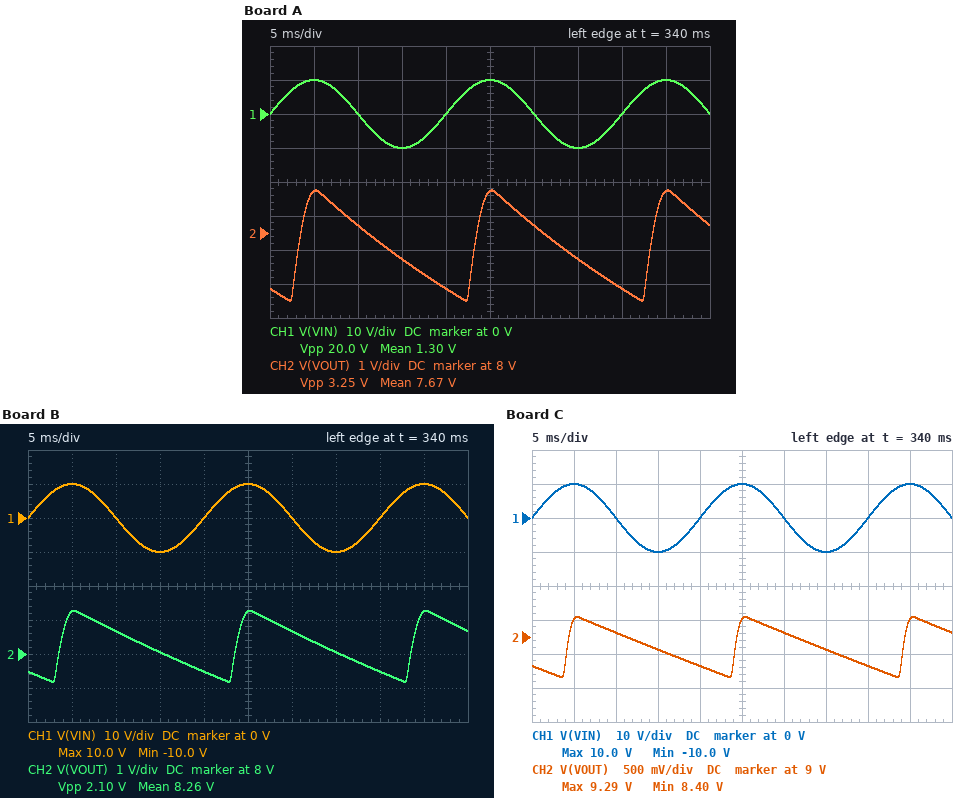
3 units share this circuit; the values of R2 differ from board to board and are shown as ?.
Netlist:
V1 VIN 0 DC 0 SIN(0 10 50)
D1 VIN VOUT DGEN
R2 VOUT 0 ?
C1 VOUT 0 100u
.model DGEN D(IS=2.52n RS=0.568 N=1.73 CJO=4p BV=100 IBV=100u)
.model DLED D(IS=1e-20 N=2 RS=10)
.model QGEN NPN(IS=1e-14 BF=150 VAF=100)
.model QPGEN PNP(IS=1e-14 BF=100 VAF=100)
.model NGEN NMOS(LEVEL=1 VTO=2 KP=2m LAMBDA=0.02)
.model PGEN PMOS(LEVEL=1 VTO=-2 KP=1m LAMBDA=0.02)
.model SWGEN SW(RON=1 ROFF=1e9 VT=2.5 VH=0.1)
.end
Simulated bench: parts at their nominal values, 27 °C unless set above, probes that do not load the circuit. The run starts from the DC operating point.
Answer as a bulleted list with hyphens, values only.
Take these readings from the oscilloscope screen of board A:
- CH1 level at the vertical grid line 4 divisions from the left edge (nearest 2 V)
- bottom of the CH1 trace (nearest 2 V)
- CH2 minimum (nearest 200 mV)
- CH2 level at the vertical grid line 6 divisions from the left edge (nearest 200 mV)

- 0 V
- -10 V
- 6.0 V
- 8.2 V
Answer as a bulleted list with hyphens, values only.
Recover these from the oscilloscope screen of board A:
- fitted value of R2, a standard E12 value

- 390 Ω
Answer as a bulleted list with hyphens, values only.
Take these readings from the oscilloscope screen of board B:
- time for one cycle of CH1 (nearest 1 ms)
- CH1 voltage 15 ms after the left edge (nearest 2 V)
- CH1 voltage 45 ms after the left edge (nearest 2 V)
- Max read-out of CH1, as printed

- 20 ms
- -10 V
- 10 V
- 10.0 V
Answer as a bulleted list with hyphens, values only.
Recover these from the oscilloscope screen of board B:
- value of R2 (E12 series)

- 680 Ω
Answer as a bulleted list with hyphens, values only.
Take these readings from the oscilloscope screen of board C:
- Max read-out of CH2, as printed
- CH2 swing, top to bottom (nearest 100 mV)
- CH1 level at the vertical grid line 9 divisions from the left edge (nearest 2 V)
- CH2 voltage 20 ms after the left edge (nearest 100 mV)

- 9.29 V
- 900 mV
- 10 V
- 8.6 V
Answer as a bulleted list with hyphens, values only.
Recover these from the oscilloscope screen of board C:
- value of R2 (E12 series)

- 1.8 kΩ
